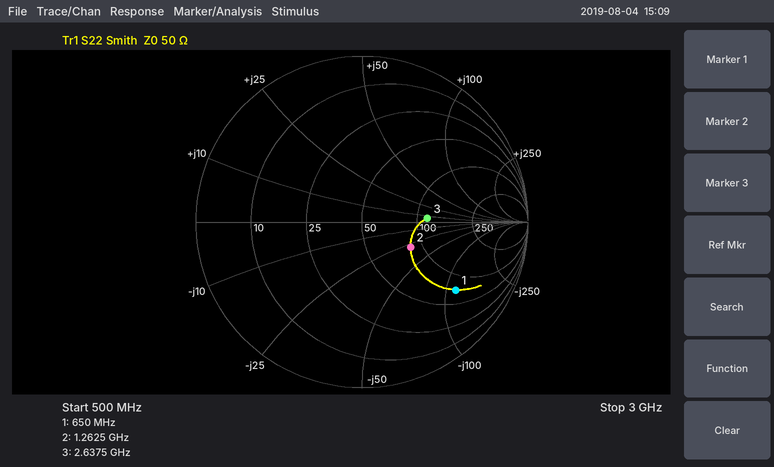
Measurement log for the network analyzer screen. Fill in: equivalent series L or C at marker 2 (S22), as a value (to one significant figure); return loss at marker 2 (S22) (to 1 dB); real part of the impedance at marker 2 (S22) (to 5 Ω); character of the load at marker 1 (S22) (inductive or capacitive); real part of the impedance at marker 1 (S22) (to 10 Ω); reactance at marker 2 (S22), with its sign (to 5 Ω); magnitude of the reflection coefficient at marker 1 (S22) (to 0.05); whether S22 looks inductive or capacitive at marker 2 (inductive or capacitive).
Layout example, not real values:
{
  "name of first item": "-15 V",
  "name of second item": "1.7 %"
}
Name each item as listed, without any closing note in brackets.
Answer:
{
  "equivalent series L or C at marker 2 (S22), as a value": "4 pF",
  "return loss at marker 2 (S22)": "10 dB",
  "real part of the impedance at marker 2 (S22)": "85 Ω",
  "character of the load at marker 1 (S22)": "capacitive",
  "real part of the impedance at marker 1 (S22)": "70 Ω",
  "reactance at marker 2 (S22), with its sign": "-30 Ω",
  "magnitude of the reflection coefficient at marker 1 (S22)": "0.70",
  "whether S22 looks inductive or capacitive at marker 2": "capacitive"
}
